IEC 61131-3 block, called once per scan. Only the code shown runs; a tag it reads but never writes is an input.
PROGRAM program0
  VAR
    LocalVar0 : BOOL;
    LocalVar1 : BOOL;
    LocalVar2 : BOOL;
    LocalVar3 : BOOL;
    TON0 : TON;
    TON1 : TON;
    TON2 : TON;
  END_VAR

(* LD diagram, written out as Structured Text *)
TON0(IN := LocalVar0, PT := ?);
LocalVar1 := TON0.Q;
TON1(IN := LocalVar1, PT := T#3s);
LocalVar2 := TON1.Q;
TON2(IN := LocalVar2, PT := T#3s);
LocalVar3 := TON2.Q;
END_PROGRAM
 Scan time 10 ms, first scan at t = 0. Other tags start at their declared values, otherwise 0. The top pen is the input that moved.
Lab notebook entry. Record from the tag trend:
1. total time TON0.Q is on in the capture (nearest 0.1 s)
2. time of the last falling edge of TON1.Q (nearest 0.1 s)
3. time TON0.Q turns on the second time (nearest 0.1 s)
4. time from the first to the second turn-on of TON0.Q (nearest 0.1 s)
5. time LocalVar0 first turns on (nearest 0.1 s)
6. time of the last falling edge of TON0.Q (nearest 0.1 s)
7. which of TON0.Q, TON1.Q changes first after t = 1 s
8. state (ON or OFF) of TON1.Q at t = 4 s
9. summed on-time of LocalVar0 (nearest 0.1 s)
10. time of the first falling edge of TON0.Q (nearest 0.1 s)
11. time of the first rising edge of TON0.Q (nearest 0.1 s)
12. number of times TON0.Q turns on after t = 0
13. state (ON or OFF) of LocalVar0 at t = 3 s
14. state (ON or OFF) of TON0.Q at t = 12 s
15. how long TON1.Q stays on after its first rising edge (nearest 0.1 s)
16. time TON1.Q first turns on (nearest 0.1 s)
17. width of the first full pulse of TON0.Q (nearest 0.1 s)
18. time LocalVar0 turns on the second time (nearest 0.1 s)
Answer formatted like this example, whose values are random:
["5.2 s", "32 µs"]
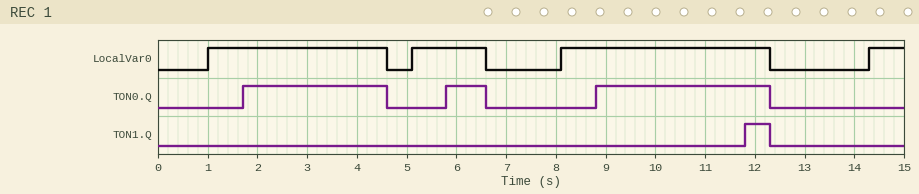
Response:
["7.2 s", "12.3 s", "5.8 s", "4.1 s", "1.0 s", "12.3 s", "TON0.Q", "OFF", "10.0 s", "4.6 s", "1.7 s", "3", "ON", "ON", "0.5 s", "11.8 s", "2.9 s", "5.1 s"]
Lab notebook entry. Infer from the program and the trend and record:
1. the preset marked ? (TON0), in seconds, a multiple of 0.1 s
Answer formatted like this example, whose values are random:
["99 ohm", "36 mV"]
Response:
["0.7 s"]
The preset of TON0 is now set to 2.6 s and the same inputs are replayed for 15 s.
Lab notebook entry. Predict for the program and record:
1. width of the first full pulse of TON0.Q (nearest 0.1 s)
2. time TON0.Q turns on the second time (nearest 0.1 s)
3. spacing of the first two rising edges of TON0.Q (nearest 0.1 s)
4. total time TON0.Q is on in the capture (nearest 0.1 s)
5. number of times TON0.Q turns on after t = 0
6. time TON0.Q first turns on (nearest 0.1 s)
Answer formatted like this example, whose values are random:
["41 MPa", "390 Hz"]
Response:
["1.0 s", "10.7 s", "7.1 s", "2.6 s", "2", "3.6 s"]
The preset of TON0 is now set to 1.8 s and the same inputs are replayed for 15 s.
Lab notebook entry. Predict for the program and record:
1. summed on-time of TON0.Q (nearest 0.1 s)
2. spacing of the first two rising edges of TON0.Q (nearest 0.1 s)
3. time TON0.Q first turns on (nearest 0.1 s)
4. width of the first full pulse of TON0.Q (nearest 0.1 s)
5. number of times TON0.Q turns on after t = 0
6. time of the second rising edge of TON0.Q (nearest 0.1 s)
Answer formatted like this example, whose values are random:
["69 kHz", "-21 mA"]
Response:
["4.2 s", "7.1 s", "2.8 s", "1.8 s", "2", "9.9 s"]
